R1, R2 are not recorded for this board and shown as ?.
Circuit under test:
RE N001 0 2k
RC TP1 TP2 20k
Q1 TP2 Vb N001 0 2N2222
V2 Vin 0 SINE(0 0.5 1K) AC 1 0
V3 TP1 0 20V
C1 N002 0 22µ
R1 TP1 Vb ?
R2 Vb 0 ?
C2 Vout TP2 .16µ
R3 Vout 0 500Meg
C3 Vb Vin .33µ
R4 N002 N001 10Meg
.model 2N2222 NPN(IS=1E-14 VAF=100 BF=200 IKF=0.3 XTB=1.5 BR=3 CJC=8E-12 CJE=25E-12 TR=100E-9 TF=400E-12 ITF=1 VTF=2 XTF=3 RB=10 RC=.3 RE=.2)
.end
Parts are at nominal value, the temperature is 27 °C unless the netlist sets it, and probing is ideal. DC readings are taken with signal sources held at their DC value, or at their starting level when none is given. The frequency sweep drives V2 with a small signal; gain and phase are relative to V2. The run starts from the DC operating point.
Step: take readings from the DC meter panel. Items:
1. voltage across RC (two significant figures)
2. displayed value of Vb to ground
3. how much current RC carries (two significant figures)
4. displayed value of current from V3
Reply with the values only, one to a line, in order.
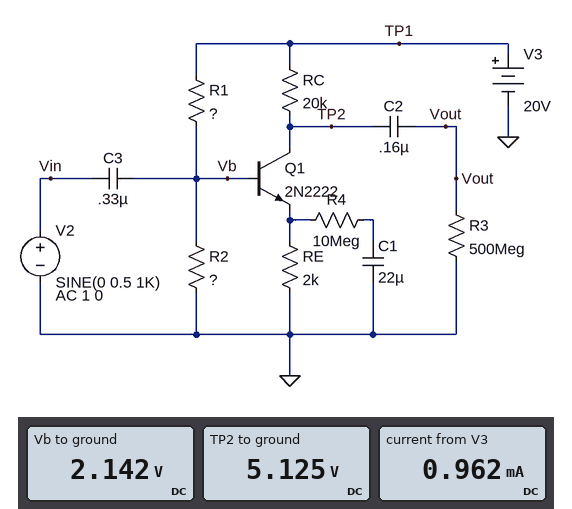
15 V
2.142 V
740 µA
0.962 mA
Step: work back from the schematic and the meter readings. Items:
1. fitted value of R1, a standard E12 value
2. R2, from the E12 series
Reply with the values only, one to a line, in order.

82 kΩ
10 kΩ
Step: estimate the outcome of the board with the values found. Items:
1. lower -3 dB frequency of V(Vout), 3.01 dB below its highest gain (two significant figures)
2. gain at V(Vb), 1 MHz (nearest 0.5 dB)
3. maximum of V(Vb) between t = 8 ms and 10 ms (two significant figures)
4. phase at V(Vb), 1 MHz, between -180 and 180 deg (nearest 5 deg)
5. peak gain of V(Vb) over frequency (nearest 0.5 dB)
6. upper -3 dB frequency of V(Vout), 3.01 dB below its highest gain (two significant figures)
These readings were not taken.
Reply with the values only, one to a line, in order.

55 Hz
0 dB
2.6 V
0 deg
0 dB
1.7 MHz
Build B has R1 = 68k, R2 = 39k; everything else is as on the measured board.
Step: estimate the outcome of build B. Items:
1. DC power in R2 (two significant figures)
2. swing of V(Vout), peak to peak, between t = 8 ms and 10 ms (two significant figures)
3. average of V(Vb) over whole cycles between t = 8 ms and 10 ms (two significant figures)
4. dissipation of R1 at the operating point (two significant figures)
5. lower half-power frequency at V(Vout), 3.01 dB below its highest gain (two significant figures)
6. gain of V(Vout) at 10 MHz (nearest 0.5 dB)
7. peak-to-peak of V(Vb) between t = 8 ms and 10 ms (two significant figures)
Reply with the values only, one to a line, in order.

200 µW
1.7 V
2.8 V
4.3 mW
330 Hz
0 dB
970 mV
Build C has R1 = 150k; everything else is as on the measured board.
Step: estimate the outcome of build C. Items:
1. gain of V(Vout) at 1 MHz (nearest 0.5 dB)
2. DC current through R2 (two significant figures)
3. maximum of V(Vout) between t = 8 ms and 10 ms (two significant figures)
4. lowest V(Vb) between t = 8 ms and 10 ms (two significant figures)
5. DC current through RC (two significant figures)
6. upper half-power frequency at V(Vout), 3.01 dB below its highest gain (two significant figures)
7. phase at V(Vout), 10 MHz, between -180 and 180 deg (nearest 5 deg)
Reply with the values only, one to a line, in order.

19.0 dB
120 µA
4.6 V
740 mV
310 µA
2.6 MHz
70 deg
